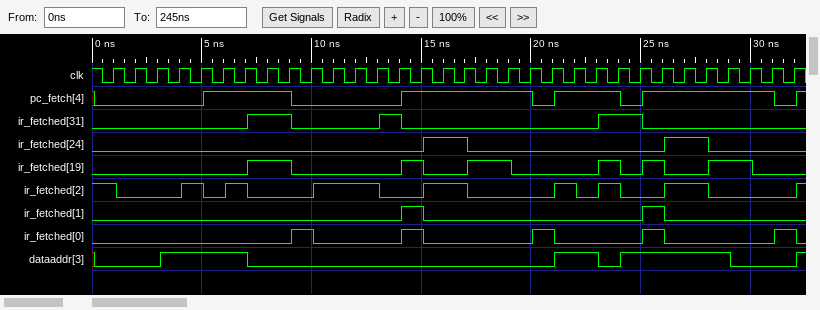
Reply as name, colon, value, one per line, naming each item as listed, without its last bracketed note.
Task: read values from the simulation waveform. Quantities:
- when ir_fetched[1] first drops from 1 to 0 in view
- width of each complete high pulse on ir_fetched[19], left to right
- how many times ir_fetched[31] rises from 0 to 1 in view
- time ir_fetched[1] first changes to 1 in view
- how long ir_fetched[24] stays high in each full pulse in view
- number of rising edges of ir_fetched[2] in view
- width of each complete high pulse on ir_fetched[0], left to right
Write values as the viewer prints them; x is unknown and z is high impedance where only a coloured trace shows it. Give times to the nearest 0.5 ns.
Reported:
when ir_fetched[1] first drops from 1 to 0 in view: 15 ns
width of each complete high pulse on ir_fetched[19], left to right: 2 ns, 1 ns, 2 ns, 1 ns, 1 ns, 2 ns
how many times ir_fetched[31] rises from 0 to 1 in view: 3
time ir_fetched[1] first changes to 1 in view: 14 ns
how long ir_fetched[24] stays high in each full pulse in view: 2 ns, 2 ns
number of rising edges of ir_fetched[2] in view: 8
width of each complete high pulse on ir_fetched[0], left to right: 1 ns, 1 ns, 1 ns, 1 ns, 1 ns
